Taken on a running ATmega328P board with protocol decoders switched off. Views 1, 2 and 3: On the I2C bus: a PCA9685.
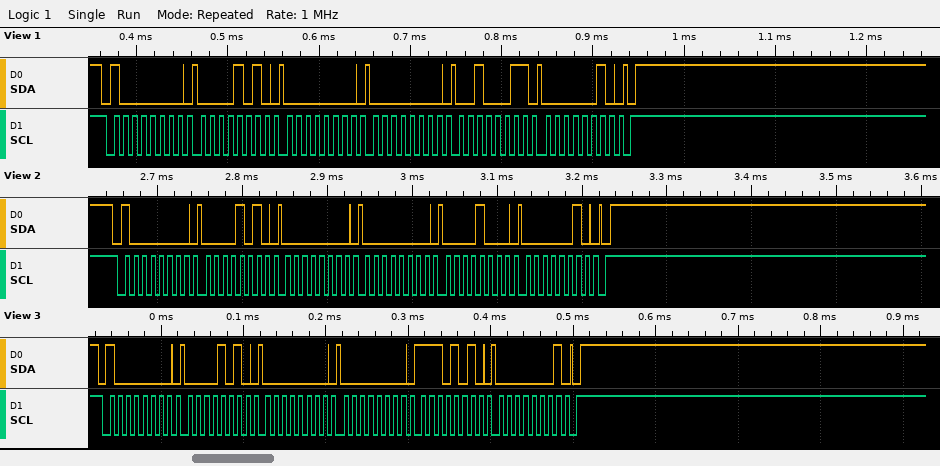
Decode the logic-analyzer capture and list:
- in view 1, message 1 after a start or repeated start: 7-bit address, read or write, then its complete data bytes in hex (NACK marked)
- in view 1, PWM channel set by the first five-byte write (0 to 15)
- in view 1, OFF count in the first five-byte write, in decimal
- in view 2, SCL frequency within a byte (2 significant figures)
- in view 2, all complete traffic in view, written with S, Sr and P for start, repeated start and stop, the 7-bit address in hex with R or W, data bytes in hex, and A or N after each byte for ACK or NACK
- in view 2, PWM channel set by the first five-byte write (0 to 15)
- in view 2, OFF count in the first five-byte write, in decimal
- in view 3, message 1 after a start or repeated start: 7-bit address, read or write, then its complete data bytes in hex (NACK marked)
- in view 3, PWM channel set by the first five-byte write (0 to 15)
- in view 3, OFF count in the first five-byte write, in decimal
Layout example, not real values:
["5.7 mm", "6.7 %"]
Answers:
["0x40 write: 0A 00 00 23 02", "1", "547", "100 kHz", "S 40W A 0A A 00 A 00 A 08 A 02 A P", "1", "520", "0x40 write: 0A 00 00 EA 01", "1", "490"]
